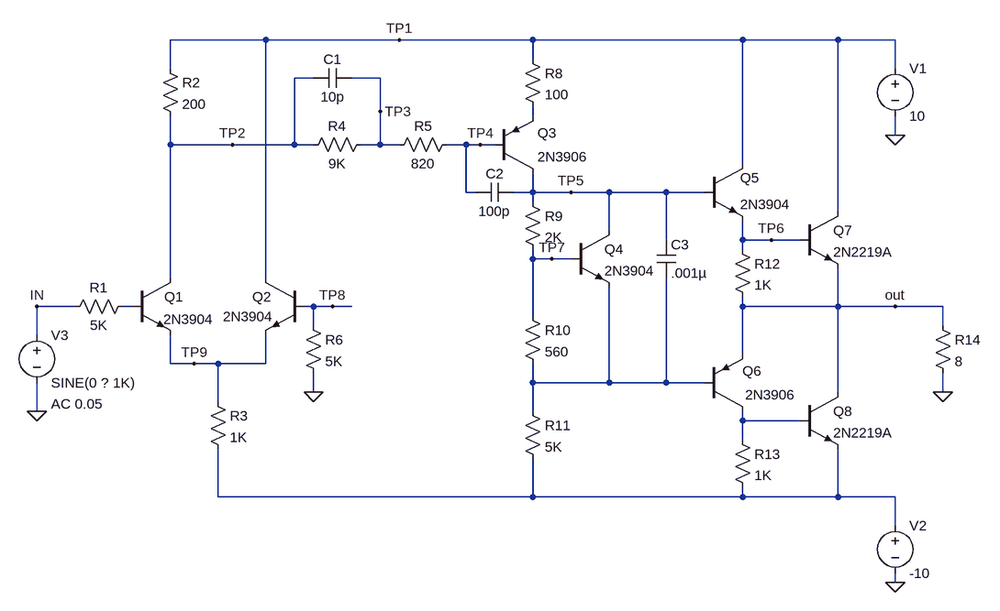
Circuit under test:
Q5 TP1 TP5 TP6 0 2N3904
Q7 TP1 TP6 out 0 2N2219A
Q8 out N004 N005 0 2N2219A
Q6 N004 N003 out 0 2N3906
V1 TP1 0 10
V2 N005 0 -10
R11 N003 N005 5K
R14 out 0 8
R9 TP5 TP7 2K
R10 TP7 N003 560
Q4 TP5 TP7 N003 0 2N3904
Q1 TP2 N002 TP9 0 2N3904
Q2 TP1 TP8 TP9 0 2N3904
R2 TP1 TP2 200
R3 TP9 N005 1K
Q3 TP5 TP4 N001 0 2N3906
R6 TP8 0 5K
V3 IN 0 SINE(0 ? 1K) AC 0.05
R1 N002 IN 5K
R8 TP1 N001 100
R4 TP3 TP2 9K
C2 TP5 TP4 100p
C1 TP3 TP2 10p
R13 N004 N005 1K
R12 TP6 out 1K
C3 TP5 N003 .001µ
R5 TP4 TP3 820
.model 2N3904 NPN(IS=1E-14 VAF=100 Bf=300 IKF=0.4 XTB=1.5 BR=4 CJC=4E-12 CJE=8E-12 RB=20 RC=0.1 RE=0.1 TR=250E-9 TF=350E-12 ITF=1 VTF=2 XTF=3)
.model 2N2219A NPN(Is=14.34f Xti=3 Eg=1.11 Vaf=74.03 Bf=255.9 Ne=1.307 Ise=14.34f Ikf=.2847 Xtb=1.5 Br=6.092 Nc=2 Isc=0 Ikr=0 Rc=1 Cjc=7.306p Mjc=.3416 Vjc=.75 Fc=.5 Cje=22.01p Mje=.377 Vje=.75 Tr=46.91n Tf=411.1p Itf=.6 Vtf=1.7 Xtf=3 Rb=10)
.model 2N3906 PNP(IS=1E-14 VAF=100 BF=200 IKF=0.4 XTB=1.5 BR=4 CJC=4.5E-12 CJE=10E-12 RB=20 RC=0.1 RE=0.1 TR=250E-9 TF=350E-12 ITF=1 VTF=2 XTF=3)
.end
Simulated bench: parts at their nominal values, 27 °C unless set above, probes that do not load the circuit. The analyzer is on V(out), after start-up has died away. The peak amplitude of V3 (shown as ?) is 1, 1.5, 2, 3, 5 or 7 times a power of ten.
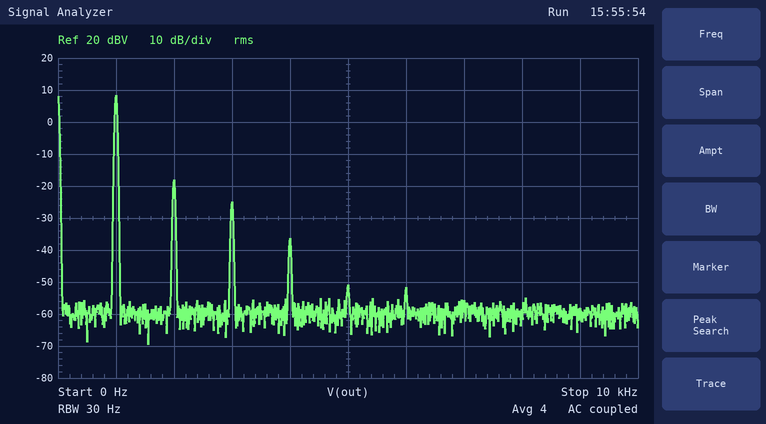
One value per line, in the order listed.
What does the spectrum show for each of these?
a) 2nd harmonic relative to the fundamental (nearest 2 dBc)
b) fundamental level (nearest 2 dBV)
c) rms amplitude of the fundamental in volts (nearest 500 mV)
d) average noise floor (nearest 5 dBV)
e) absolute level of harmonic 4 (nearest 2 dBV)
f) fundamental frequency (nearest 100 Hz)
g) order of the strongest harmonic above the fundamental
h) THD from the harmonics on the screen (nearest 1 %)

-26 dBc
8 dBV
2.5 V
-60 dBV
-36 dBV
1.0 kHz
2
5 %
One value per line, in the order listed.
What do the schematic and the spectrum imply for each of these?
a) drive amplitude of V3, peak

30 mV
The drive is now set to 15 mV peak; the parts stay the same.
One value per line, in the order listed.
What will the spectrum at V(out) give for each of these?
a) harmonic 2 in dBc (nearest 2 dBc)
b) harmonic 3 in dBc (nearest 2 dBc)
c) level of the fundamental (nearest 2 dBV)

-38 dBc
-48 dBc
2 dBV
